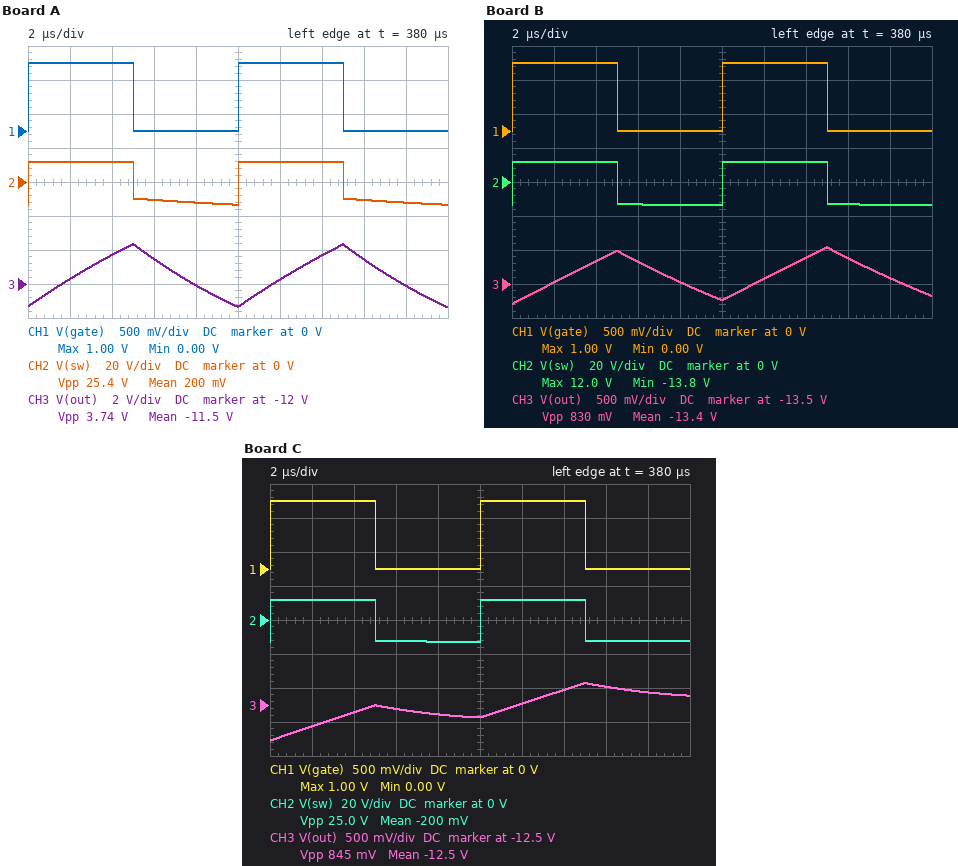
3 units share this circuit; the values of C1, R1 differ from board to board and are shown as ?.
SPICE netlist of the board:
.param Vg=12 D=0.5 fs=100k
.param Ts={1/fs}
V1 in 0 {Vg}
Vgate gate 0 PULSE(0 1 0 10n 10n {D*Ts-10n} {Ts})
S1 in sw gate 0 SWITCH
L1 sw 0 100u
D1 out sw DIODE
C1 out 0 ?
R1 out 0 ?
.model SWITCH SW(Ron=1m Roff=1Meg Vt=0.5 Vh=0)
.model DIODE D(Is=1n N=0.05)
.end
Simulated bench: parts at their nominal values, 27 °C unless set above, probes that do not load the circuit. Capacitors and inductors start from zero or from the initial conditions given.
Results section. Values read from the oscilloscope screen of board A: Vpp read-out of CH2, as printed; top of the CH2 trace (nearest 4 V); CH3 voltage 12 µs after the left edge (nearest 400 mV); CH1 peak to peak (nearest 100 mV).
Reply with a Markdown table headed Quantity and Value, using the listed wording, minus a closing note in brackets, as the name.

| Quantity | Value |
|---|---|
| Vpp read-out of CH2, as printed | 25.4 V |
| top of the CH2 trace | 12 V |
| CH3 voltage 12 µs after the left edge | -11.6 V |
| CH1 peak to peak | 1.0 V |
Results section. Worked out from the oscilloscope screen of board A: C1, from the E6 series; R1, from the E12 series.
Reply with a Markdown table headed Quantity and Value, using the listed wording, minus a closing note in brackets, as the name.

| Quantity | Value |
|---|---|
| C1, from the E6 series | 4.7 µF |
| R1, from the E12 series | 3.3 Ω |
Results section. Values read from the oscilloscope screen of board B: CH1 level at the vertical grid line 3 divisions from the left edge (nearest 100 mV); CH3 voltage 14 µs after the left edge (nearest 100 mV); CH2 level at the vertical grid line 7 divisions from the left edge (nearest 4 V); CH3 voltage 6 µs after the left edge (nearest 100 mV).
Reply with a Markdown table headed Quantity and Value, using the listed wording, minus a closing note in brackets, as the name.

| Quantity | Value |
|---|---|
| CH1 level at the vertical grid line 3 divisions from the left edge | 0 V |
| CH3 voltage 14 µs after the left edge | -13.1 V |
| CH2 level at the vertical grid line 7 divisions from the left edge | 12 V |
| CH3 voltage 6 µs after the left edge | -13.2 V |
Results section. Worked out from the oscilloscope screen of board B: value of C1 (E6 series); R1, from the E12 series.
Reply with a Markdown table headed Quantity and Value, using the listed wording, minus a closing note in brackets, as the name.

| Quantity | Value |
|---|---|
| value of C1 | 22 µF |
| R1, from the E12 series | 3.9 Ω |
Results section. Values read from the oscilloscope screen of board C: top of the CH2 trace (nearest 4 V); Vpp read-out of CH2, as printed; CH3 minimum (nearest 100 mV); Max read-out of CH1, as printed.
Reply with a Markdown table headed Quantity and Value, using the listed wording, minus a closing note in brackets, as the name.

| Quantity | Value |
|---|---|
| top of the CH2 trace | 12 V |
| Vpp read-out of CH2, as printed | 25.0 V |
| CH3 minimum | -13.0 V |
| Max read-out of CH1, as printed | 1.00 V |
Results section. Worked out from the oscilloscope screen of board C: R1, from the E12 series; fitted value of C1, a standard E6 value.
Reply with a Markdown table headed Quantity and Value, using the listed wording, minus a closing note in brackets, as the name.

| Quantity | Value |
|---|---|
| R1, from the E12 series | 8.2 Ω |
| fitted value of C1, a standard E6 value | 15 µF |
